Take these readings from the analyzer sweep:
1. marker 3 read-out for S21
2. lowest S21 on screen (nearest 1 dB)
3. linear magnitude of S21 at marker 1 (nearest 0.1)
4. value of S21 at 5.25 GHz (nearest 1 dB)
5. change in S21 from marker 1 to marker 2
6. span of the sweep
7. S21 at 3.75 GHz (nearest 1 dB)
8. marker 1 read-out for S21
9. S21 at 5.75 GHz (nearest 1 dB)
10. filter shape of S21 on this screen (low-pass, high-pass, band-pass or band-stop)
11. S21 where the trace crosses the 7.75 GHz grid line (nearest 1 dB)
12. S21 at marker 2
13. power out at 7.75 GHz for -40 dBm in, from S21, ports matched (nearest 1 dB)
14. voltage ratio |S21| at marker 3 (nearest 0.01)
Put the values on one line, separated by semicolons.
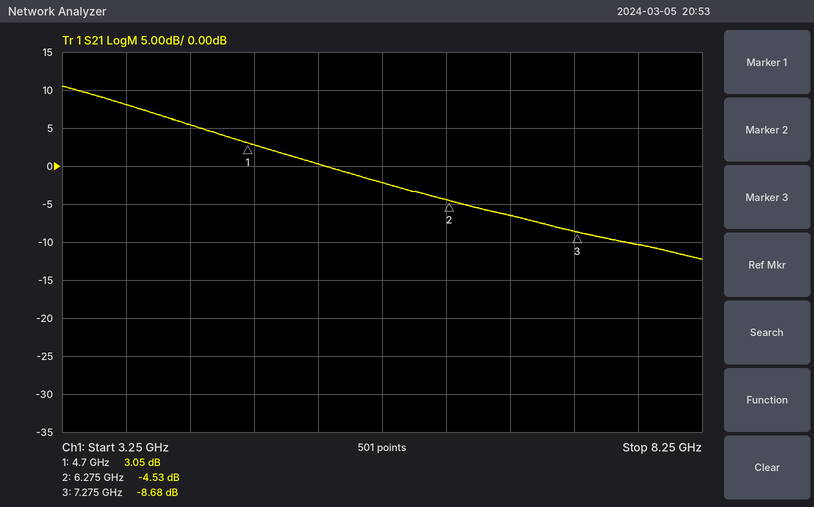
-8.68 dB; -12 dB; 1.4; 0 dB; -7.58 dB; 5 GHz; 8 dB; 3.05 dB; -2 dB; low-pass; -10 dB; -4.53 dB; -50 dBm; 0.37
